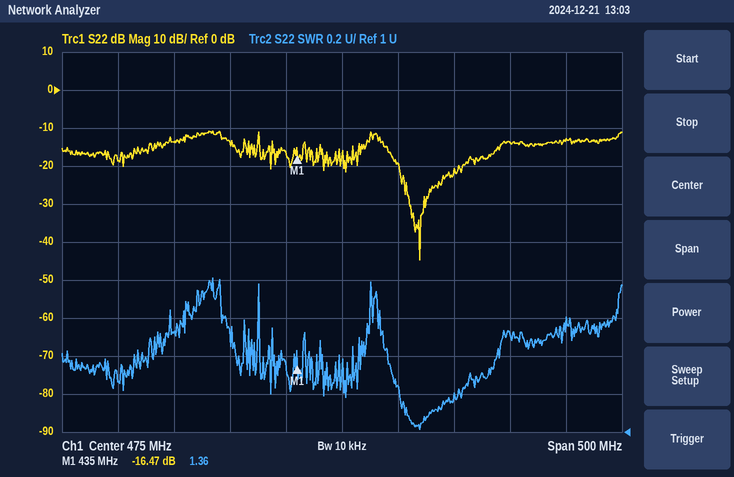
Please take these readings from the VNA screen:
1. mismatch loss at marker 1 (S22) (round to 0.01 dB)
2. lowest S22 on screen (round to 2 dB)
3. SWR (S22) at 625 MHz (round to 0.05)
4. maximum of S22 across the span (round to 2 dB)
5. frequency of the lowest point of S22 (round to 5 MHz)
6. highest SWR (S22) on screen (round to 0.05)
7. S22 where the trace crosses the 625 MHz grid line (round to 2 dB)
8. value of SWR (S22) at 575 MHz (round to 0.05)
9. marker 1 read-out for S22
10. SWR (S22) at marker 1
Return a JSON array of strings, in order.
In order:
["0.10 dB", "-44 dB", "1.50", "-10 dB", "545 MHz", "1.80", "-14 dB", "1.20", "-16.47 dB", "1.36"]
